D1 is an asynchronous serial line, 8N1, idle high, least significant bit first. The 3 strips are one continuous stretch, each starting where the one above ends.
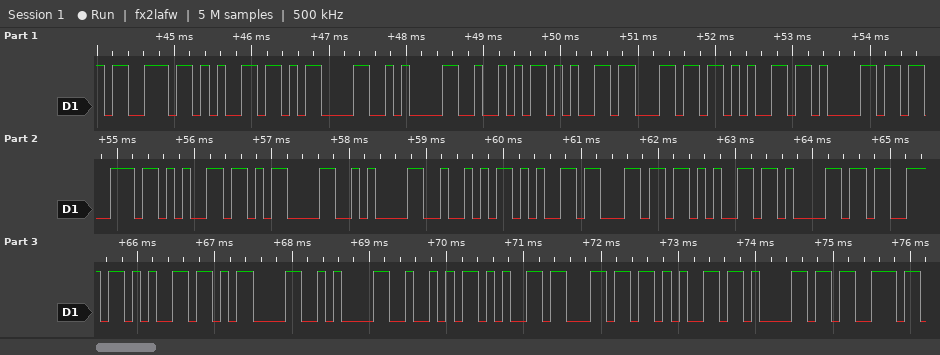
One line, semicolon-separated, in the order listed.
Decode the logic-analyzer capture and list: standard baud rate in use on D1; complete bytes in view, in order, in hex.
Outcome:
9600 baud; 73 65 0D 0A 52 65 6C 65 61 73 65 0D 0A 52 65 6C 65 61 73 65 0D 0A 52 65 6C 65 61 73
